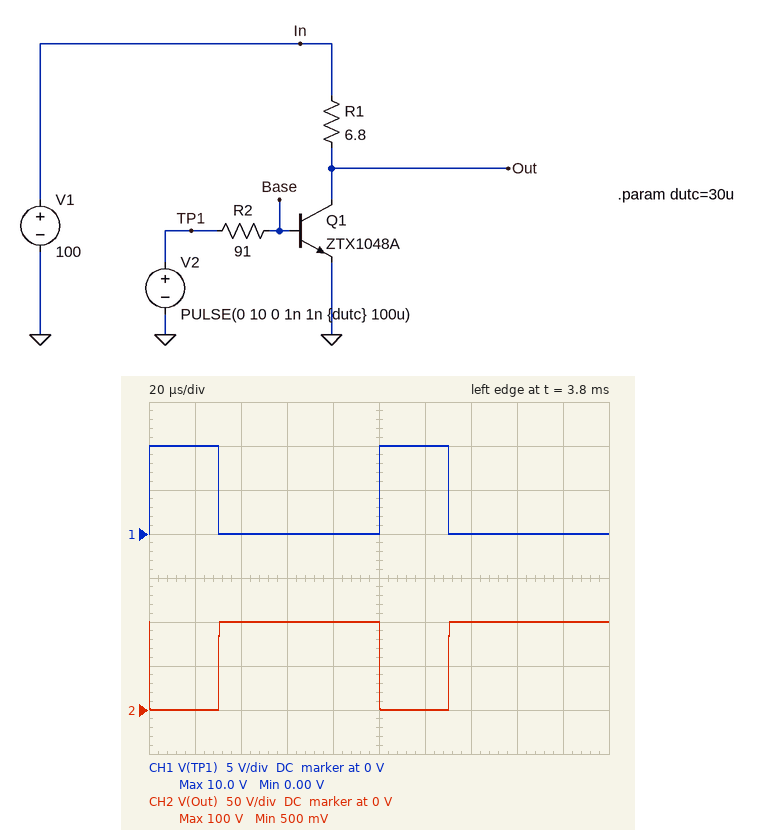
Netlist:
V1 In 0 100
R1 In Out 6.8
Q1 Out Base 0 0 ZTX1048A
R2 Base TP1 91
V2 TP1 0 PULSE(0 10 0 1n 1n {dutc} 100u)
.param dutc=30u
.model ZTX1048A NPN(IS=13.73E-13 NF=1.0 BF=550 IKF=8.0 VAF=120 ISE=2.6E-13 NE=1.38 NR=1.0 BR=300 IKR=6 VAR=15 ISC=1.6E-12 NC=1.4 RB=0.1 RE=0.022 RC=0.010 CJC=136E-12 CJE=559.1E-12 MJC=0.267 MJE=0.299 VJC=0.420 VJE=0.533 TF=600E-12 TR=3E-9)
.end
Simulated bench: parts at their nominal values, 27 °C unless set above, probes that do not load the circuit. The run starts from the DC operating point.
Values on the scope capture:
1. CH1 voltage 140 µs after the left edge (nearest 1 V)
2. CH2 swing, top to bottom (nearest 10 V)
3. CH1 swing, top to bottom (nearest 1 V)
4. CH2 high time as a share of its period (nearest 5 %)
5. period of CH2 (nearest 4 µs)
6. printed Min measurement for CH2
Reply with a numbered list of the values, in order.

1. 0 V
2. 100 V
3. 10 V
4. 70 %
5. 100 µs
6. 500 mV
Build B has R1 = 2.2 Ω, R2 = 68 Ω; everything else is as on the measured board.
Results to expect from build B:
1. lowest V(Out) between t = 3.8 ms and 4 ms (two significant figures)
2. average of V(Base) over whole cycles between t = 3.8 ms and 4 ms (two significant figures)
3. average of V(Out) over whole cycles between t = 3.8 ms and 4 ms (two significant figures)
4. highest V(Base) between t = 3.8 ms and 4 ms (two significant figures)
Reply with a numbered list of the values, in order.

1. 44 V
2. 420 mV
3. 83 V
4. 1.4 V
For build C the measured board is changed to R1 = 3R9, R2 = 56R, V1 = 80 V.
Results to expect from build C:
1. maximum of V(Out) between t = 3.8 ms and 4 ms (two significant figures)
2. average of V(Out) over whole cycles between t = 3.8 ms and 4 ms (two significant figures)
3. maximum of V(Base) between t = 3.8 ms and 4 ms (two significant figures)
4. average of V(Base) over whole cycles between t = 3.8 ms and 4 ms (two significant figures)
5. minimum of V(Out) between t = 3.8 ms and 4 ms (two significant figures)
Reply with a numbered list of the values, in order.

1. 80 V
2. 56 V
3. 1.3 V
4. 390 mV
5. 770 mV
